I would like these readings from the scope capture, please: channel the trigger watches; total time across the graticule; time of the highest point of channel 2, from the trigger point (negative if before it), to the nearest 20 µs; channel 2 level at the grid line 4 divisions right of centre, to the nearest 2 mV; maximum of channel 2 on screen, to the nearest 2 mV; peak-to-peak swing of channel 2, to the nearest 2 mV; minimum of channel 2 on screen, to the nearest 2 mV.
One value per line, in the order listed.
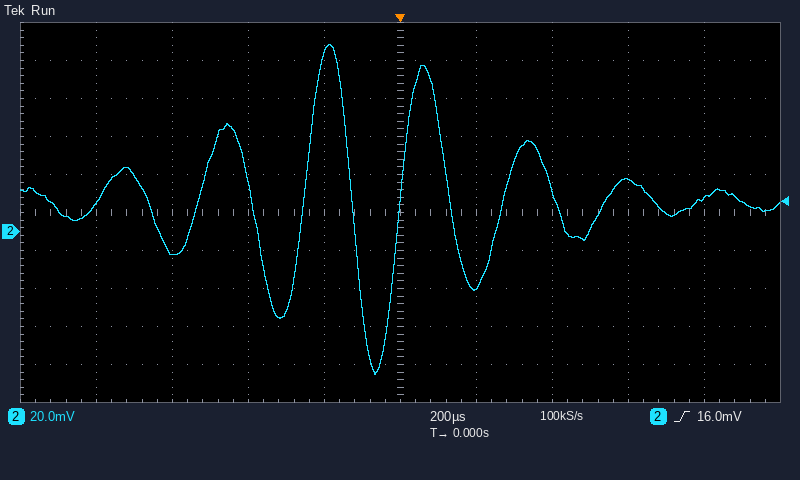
channel 2
2 ms
-180 µs
18 mV
98 mV
174 mV
-76 mV
